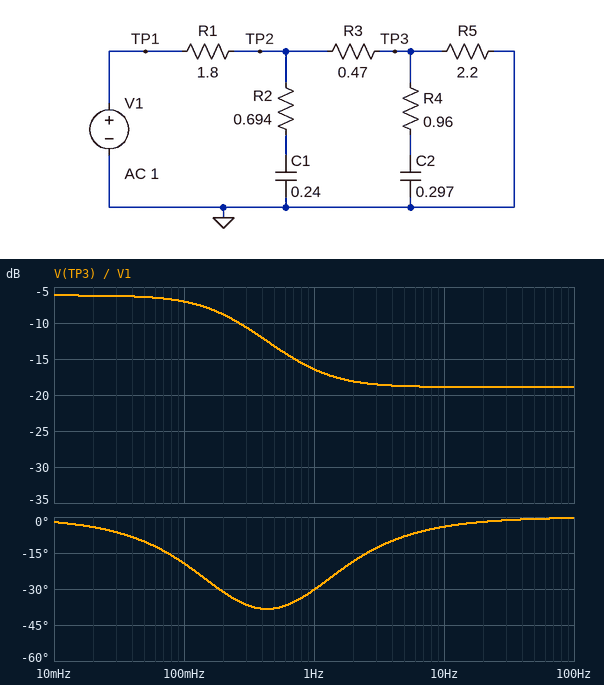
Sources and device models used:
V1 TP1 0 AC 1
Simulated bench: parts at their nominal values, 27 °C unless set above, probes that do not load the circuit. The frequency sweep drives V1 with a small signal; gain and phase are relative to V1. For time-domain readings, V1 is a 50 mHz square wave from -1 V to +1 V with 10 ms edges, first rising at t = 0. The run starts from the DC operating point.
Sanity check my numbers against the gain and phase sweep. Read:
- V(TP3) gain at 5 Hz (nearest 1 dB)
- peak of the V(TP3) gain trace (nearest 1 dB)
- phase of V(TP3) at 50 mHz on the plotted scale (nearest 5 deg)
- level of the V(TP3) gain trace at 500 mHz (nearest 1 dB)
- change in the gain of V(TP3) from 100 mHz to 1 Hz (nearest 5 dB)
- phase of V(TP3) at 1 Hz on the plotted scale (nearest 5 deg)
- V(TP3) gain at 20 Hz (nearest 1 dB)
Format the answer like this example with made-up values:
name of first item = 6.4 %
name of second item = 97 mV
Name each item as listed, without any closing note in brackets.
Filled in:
V(TP3) gain at 5 Hz = -19 dB
peak of the V(TP3) gain trace = -6 dB
phase of V(TP3) at 50 mHz on the plotted scale = -10 deg
level of the V(TP3) gain trace at 500 mHz = -13 dB
change in the gain of V(TP3) from 100 mHz to 1 Hz = -10 dB
phase of V(TP3) at 1 Hz on the plotted scale = -30 deg
V(TP3) gain at 20 Hz = -19 dB
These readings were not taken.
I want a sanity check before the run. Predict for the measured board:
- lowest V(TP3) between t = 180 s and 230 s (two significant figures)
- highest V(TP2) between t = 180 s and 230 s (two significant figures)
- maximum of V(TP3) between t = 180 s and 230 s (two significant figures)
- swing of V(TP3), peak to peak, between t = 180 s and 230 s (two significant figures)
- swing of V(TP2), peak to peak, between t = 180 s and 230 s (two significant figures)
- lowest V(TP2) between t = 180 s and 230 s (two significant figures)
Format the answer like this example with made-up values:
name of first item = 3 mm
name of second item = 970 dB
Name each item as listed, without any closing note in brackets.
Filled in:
lowest V(TP3) between t = 180 s and 230 s = -490 mV
highest V(TP2) between t = 180 s and 230 s = 600 mV
maximum of V(TP3) between t = 180 s and 230 s = 490 mV
swing of V(TP3), peak to peak, between t = 180 s and 230 s = 980 mV
swing of V(TP2), peak to peak, between t = 180 s and 230 s = 1.2 V
lowest V(TP2) between t = 180 s and 230 s = -600 mV
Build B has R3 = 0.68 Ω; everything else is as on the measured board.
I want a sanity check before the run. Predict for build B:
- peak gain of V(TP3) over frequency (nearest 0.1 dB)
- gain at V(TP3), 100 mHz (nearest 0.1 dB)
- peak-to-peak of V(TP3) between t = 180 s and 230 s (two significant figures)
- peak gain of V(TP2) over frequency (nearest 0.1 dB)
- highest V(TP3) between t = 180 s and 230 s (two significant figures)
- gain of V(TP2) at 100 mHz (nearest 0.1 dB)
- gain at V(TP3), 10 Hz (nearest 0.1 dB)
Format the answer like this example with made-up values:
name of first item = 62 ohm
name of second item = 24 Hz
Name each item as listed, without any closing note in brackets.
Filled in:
peak gain of V(TP3) over frequency = -6.6 dB
gain at V(TP3), 100 mHz = -7.4 dB
peak-to-peak of V(TP3) between t = 180 s and 230 s = 940 mV
peak gain of V(TP2) over frequency = -4.2 dB
highest V(TP3) between t = 180 s and 230 s = 470 mV
gain of V(TP2) at 100 mHz = -4.9 dB
gain at V(TP3), 10 Hz = -19.9 dB
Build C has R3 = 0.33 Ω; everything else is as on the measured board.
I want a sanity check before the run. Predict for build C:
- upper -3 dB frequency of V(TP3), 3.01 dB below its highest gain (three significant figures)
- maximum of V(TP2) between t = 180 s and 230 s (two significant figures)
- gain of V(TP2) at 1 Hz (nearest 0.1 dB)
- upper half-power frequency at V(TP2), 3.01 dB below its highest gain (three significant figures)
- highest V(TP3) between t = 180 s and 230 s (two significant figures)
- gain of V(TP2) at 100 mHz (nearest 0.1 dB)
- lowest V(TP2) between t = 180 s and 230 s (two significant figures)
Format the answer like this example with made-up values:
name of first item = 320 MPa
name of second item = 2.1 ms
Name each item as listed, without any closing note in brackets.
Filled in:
upper -3 dB frequency of V(TP3), 3.01 dB below its highest gain = 223 mHz
maximum of V(TP2) between t = 180 s and 230 s = 580 mV
gain of V(TP2) at 1 Hz = -12.7 dB
upper half-power frequency at V(TP2), 3.01 dB below its highest gain = 249 mHz
highest V(TP3) between t = 180 s and 230 s = 510 mV
gain of V(TP2) at 100 mHz = -5.4 dB
lowest V(TP2) between t = 180 s and 230 s = -580 mV
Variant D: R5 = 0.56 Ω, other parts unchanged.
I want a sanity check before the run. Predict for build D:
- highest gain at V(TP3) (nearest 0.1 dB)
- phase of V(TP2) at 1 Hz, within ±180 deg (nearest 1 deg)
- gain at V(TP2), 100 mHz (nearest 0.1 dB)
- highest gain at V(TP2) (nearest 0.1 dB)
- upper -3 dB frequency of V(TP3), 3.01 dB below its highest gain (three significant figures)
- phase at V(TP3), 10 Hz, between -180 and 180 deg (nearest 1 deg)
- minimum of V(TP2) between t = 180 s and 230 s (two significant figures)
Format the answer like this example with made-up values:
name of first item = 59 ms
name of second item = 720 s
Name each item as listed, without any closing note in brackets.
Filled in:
highest gain at V(TP3) = -14.1 dB
phase of V(TP2) at 1 Hz, within ±180 deg = -18 deg
gain at V(TP2), 100 mHz = -9.0 dB
highest gain at V(TP2) = -8.8 dB
upper -3 dB frequency of V(TP3), 3.01 dB below its highest gain = 405 mHz
phase at V(TP3), 10 Hz, between -180 and 180 deg = -3 deg
minimum of V(TP2) between t = 180 s and 230 s = -360 mV
